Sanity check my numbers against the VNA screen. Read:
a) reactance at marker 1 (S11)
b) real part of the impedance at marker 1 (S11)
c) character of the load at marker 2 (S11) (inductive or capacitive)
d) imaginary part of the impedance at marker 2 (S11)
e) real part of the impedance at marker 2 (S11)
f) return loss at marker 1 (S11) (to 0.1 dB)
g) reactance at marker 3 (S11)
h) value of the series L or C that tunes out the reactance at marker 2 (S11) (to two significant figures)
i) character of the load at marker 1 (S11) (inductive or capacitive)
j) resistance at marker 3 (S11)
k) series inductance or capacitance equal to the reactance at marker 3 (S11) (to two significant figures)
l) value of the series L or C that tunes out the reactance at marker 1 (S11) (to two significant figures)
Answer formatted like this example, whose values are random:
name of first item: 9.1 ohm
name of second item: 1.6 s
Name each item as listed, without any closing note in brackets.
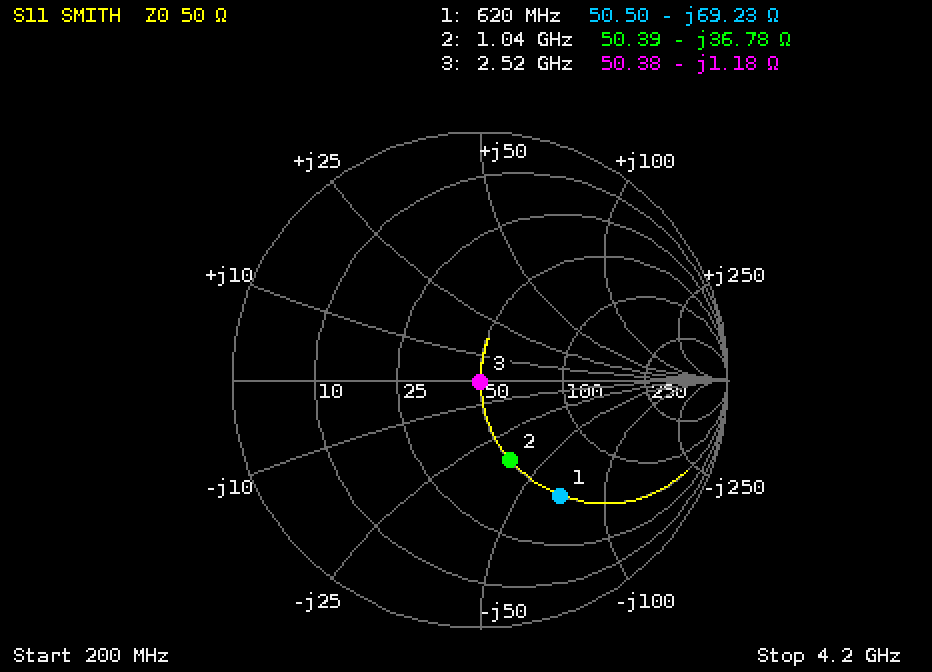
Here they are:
reactance at marker 1: -69.23 Ω
real part of the impedance at marker 1: 50.50 Ω
character of the load at marker 2 (S11): capacitive
imaginary part of the impedance at marker 2: -36.78 Ω
real part of the impedance at marker 2: 50.39 Ω
return loss at marker 1 (S11): 4.9 dB
reactance at marker 3: -1.18 Ω
value of the series L or C that tunes out the reactance at marker 2 (S11): 5.6 nH
character of the load at marker 1 (S11): capacitive
resistance at marker 3: 50.38 Ω
series inductance or capacitance equal to the reactance at marker 3 (S11): 54 pF
value of the series L or C that tunes out the reactance at marker 1 (S11): 18 nH
